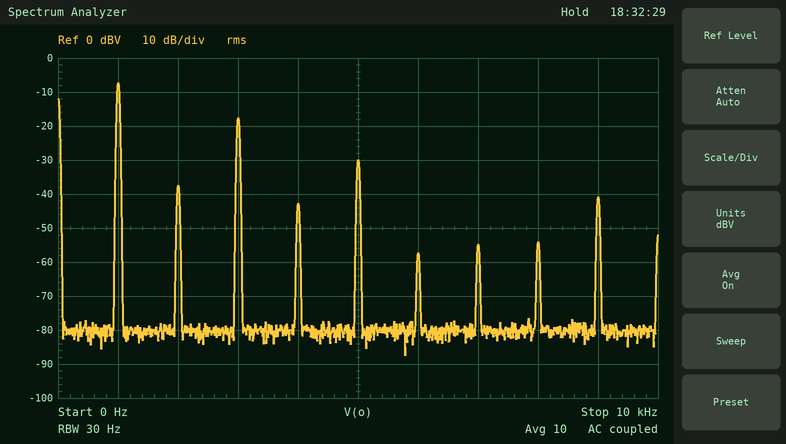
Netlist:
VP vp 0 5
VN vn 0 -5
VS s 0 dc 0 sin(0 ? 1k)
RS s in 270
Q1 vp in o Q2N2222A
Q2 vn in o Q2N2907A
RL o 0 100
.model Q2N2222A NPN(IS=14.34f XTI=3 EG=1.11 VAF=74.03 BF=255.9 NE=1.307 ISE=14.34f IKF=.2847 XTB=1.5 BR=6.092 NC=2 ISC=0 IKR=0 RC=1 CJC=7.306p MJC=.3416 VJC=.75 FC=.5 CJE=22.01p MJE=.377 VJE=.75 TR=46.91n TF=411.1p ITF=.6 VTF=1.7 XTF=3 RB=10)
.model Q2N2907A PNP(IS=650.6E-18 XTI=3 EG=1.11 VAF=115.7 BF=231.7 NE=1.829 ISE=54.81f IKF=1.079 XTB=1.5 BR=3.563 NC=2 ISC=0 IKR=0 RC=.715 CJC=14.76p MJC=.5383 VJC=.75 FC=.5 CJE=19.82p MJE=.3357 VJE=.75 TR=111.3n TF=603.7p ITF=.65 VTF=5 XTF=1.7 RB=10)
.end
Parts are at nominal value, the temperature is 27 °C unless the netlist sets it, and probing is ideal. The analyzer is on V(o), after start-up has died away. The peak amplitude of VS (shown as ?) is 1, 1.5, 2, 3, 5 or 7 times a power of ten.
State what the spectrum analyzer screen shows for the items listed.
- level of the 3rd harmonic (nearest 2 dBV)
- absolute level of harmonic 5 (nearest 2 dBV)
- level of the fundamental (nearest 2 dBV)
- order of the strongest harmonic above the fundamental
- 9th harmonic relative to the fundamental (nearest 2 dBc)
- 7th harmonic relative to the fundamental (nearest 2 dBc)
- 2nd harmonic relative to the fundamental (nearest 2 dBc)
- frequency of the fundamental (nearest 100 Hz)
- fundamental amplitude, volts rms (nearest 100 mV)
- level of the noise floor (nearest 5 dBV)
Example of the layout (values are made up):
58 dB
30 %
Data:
-18 dBV
-30 dBV
-8 dBV
3
-34 dBc
-48 dBc
-30 dBc
1.0 kHz
400 mV
-80 dBV
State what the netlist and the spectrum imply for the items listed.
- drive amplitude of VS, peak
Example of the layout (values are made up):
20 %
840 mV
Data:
1.5 V
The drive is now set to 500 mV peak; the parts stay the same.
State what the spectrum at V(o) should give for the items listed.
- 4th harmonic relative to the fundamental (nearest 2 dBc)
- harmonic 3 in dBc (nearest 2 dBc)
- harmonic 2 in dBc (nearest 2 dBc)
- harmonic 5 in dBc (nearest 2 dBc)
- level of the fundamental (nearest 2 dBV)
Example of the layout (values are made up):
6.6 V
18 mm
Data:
-4 dBc
-2 dBc
-2 dBc
-6 dBc
-86 dBV
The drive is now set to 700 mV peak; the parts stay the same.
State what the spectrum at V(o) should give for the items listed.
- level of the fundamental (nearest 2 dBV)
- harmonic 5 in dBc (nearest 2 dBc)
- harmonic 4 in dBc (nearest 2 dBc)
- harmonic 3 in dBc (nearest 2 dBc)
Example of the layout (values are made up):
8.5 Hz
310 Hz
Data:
-38 dBV
-8 dBc
-10 dBc
-2 dBc
